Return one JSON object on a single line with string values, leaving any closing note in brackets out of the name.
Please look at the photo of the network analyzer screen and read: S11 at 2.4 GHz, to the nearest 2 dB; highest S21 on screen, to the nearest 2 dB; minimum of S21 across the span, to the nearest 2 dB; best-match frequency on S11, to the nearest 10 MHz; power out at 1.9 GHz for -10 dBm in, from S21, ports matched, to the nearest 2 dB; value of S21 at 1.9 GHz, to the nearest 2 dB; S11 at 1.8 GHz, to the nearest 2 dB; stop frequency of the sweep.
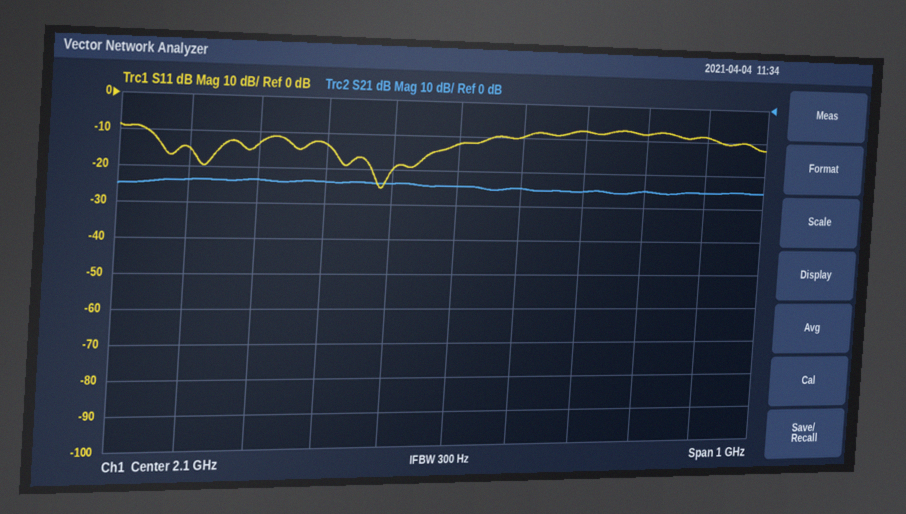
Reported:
{"S11 at 2.4 GHz, to the nearest 2 dB": "-8 dB", "highest S21 on screen, to the nearest 2 dB": "-24 dB", "minimum of S21 across the span, to the nearest 2 dB": "-26 dB", "best-match frequency on S11, to the nearest 10 MHz": "1.98 GHz", "power out at 1.9 GHz for -10 dBm in, from S21, ports matched, to the nearest 2 dB": "-34 dBm", "value of S21 at 1.9 GHz, to the nearest 2 dB": "-24 dB", "S11 at 1.8 GHz, to the nearest 2 dB": "-14 dB", "stop frequency of the sweep": "2.6 GHz"}
